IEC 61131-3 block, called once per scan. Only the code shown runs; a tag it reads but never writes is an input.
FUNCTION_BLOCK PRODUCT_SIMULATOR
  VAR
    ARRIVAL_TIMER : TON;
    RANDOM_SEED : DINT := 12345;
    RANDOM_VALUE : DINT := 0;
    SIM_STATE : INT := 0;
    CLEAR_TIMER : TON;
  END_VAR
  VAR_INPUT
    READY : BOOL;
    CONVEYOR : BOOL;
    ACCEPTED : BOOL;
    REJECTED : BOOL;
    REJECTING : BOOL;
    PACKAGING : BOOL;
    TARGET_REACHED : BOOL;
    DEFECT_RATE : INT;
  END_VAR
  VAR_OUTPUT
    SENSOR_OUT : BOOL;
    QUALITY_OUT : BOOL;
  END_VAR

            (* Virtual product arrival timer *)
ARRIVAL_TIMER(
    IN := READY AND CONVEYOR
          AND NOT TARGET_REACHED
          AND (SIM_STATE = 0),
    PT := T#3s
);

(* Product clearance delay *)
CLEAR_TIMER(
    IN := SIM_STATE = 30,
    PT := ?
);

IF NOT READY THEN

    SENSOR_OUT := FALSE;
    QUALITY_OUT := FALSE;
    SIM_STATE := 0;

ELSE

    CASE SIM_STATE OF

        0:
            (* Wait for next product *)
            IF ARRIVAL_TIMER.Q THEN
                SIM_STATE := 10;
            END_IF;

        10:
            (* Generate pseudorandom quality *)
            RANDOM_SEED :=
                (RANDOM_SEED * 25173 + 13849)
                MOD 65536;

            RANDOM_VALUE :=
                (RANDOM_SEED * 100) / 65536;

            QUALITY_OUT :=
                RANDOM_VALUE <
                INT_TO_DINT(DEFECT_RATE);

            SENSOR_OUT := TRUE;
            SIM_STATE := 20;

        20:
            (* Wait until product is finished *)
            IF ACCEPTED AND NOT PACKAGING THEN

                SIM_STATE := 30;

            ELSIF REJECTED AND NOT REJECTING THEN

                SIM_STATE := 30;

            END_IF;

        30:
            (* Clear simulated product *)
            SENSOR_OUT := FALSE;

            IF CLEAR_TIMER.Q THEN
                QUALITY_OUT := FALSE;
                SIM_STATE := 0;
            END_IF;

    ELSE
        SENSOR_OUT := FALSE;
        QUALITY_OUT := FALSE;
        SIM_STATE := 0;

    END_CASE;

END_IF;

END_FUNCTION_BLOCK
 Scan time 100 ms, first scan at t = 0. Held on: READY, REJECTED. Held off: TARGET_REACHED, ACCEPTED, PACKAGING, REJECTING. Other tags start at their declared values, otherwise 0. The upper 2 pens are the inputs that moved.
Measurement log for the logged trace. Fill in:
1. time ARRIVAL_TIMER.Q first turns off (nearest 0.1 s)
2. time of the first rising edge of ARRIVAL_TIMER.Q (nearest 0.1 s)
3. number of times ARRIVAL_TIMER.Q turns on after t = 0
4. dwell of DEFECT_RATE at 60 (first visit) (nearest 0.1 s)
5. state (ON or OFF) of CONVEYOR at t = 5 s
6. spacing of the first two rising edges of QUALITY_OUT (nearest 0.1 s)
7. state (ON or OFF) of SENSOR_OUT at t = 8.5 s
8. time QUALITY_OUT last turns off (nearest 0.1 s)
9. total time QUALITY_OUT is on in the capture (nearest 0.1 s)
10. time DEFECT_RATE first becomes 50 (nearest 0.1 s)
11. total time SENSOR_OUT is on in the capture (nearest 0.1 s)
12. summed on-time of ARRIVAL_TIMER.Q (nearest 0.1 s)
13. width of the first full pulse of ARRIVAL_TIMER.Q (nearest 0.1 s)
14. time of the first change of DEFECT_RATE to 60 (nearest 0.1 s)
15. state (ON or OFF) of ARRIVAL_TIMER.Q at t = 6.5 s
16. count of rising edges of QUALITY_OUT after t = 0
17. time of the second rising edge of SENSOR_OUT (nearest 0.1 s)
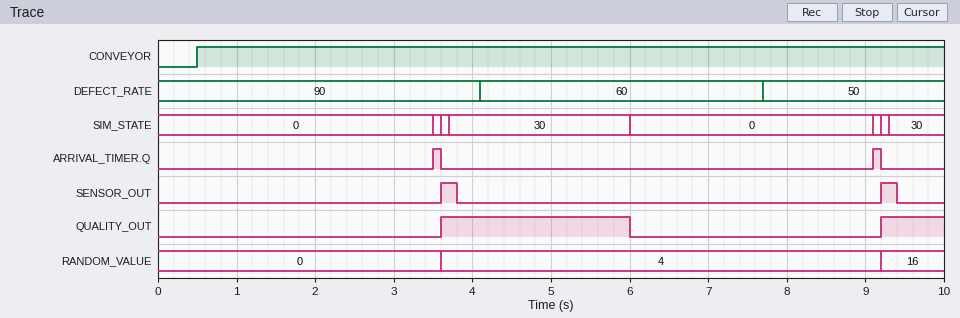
3.6 s
3.5 s
2
3.6 s
ON
5.6 s
OFF
6.0 s
3.2 s
7.7 s
0.4 s
0.2 s
0.1 s
4.1 s
OFF
2
9.2 s
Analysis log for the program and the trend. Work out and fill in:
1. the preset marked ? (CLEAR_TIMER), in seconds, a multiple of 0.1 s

2.2 s
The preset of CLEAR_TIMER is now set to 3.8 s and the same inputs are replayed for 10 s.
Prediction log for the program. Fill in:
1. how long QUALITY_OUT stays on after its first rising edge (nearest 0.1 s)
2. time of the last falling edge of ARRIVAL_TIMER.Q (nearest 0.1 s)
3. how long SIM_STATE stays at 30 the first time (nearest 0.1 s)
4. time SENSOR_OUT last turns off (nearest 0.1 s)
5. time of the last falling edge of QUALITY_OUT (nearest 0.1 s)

4.0 s
3.6 s
3.9 s
3.8 s
7.6 s
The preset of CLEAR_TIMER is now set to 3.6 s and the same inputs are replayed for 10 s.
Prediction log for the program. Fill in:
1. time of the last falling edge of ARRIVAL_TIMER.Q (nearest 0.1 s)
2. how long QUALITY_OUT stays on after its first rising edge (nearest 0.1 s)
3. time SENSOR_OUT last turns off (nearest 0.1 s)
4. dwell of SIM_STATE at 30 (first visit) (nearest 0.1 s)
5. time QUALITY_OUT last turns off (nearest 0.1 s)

3.6 s
3.8 s
3.8 s
3.7 s
7.4 s
